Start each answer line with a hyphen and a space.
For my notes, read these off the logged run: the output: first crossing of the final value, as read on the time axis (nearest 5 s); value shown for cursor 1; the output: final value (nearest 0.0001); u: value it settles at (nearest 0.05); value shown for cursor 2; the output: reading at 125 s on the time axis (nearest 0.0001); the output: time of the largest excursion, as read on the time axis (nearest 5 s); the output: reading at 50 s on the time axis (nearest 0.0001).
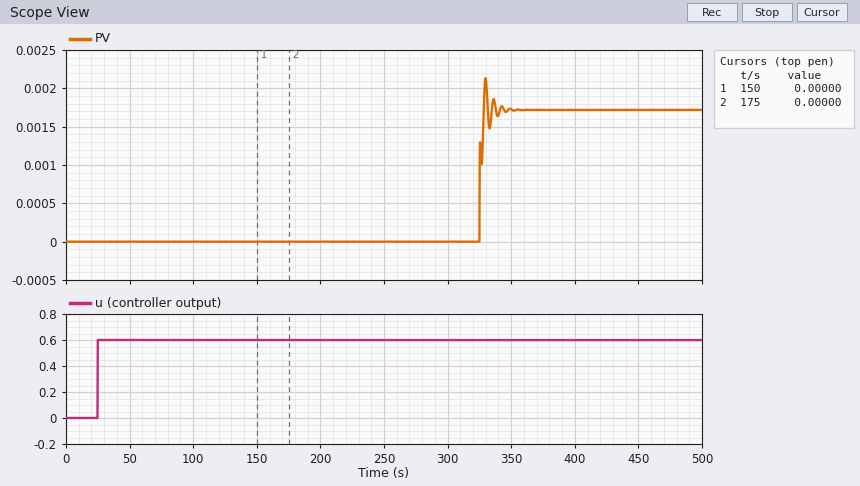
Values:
- 330 s
- 0.00000
- 0.0017
- 0.60
- 0.00000
- 0.0000
- 330 s
- 0.0000
